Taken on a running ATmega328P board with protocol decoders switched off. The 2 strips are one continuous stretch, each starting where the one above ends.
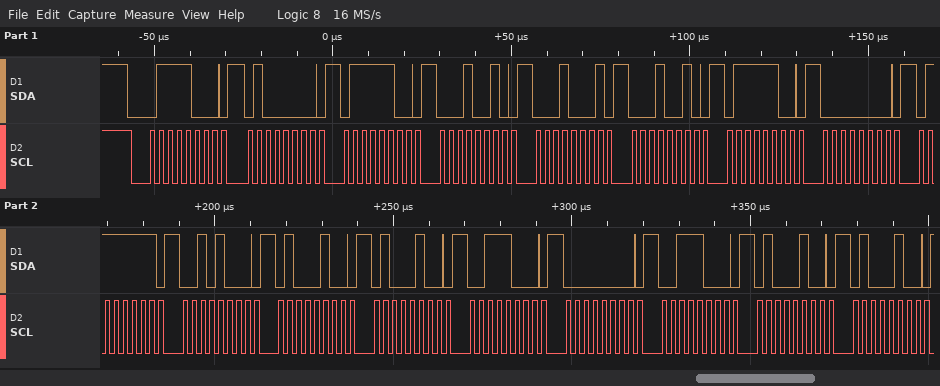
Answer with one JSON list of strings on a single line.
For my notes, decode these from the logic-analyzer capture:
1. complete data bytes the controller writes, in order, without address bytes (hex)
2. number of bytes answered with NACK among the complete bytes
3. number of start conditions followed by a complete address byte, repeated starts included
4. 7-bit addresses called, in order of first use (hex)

["40 7C 12 11 12 7C 00 7F 28 44 44 38 00 38 44 44", "0", "1", "0x3C"]
